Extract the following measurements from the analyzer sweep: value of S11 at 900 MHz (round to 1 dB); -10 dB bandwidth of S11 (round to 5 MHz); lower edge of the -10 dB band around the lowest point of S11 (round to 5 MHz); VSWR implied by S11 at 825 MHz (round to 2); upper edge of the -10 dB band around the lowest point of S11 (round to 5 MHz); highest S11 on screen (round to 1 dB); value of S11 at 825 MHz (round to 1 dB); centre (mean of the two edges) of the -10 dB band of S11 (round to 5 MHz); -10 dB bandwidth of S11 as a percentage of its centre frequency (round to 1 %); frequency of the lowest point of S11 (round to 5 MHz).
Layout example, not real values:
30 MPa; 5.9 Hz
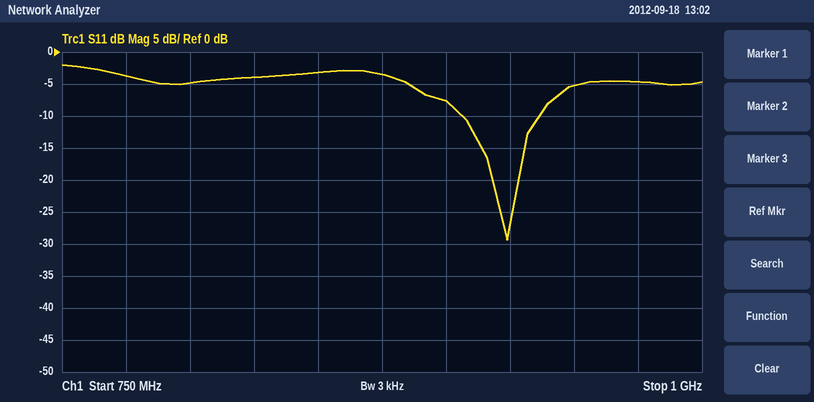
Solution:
-8 dB; 30 MHz; 905 MHz; 4; 935 MHz; -2 dB; -4 dB; 920 MHz; 3 %; 925 MHz
